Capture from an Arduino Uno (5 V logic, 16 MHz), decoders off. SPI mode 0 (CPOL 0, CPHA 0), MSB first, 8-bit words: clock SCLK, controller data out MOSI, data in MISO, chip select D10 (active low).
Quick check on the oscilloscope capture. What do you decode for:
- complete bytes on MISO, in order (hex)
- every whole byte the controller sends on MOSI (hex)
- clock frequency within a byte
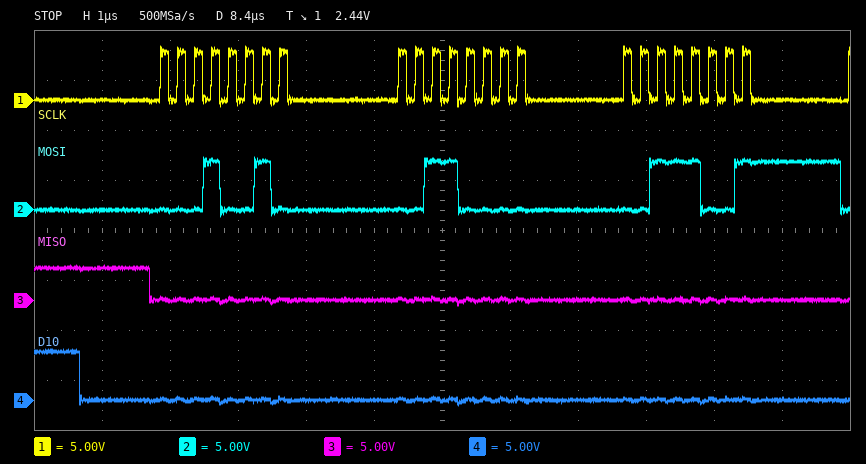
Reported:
00 00 00
12 30 39
4 MHz
